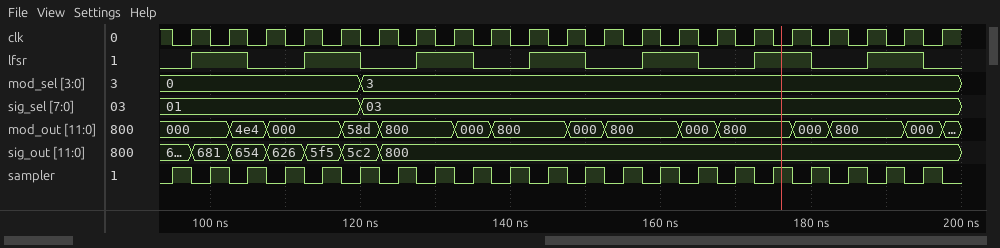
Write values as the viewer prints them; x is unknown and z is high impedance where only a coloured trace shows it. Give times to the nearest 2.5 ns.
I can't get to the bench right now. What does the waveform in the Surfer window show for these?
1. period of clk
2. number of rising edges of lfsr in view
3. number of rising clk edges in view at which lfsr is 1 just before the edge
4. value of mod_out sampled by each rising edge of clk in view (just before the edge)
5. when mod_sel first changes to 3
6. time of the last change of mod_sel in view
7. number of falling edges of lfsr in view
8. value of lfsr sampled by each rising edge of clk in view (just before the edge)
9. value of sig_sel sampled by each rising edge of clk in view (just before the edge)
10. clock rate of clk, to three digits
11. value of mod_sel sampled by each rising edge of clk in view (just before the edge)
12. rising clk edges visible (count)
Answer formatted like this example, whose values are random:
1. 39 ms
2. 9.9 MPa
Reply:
1. 5 ns
2. 7
3. 7
4. 000, 000, 4e4, 000, 000, 58d, 800, 800, 000, 800, 800, 000, 800, 800, 000, 800, 800, 000, 800, 800, 000
5. 120 ns
6. 120 ns
7. 7
8. 0 1 0 0 1 0 0 1 0 0 1 0 0 1 0 0 1 0 0 1 0
9. 01, 01, 01, 01, 01, 03, 03, 03, 03, 03, 03, 03, 03, 03, 03, 03, 03, 03, 03, 03, 03
10. 200 MHz
11. 0, 0, 0, 0, 0, 3, 3, 3, 3, 3, 3, 3, 3, 3, 3, 3, 3, 3, 3, 3, 3
12. 21
